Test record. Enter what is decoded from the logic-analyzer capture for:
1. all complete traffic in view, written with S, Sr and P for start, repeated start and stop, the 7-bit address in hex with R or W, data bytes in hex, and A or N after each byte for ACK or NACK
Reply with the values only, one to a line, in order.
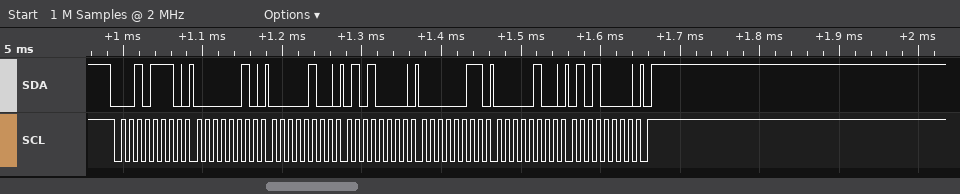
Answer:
S 17W A 02 A 04 A 50 A 03 A 04 A 50 A P
